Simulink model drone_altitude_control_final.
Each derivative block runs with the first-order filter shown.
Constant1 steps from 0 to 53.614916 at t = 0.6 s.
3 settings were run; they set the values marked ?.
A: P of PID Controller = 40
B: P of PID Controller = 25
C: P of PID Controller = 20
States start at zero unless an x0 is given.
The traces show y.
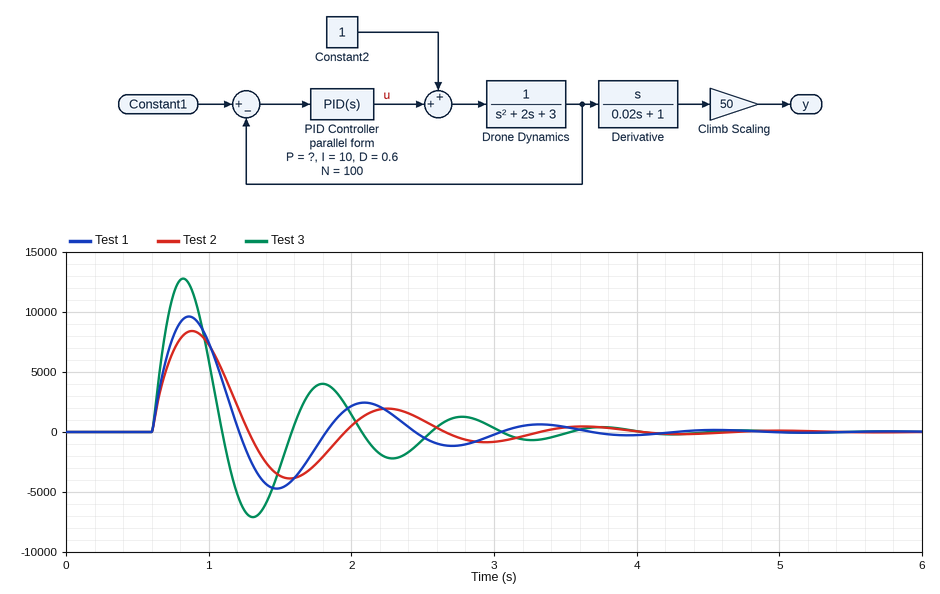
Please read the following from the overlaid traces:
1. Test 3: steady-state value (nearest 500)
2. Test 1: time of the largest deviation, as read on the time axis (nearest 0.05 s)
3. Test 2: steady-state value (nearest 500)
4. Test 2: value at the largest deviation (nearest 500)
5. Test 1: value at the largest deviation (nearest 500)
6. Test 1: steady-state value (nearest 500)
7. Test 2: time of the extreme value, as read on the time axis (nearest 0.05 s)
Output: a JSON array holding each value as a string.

["0", "0.85 s", "0", "8500", "9500", "0", "0.90 s"]
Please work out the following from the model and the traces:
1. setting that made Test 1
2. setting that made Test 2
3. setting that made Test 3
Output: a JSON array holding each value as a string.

["B", "C", "A"]
